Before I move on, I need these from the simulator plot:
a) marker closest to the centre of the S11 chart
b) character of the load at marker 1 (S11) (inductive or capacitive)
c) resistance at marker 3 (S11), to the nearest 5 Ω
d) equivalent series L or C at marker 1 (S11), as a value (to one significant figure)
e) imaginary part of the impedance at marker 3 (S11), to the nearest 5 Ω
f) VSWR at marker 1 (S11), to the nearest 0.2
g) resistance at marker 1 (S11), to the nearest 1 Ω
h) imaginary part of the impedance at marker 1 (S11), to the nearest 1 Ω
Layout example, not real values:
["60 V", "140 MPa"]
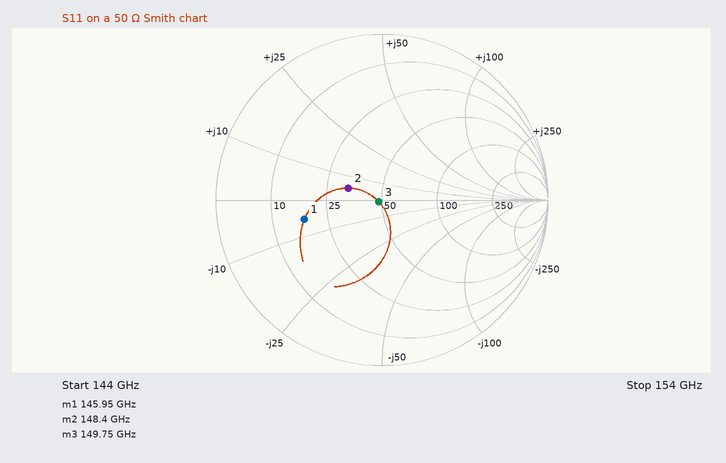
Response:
["marker 3", "capacitive", "50 Ω", "200 fF", "0 Ω", "2.8", "18 Ω", "-5 Ω"]
